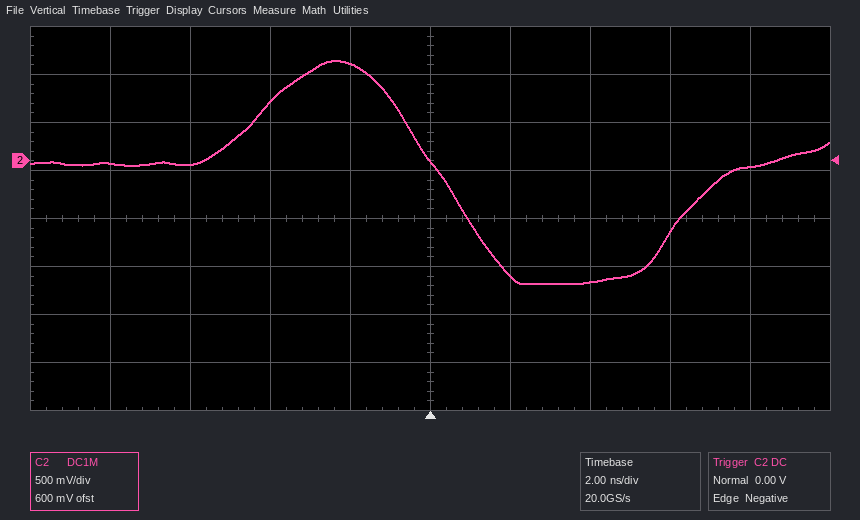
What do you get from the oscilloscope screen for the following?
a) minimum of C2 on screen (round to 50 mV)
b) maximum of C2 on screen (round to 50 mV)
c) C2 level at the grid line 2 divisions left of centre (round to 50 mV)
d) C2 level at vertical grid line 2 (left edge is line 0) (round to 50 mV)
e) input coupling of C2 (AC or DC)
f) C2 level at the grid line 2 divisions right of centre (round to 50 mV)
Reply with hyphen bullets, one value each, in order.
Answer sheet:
- -1.30 V
- 1.05 V
- 600 mV
- -50 mV
- DC
- -1.25 V
